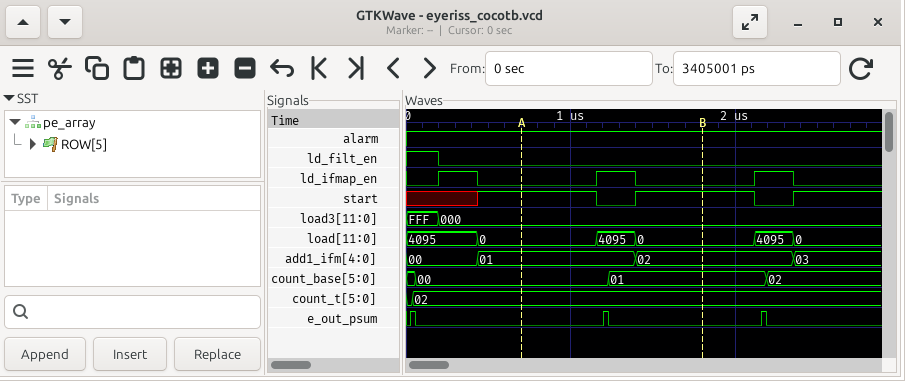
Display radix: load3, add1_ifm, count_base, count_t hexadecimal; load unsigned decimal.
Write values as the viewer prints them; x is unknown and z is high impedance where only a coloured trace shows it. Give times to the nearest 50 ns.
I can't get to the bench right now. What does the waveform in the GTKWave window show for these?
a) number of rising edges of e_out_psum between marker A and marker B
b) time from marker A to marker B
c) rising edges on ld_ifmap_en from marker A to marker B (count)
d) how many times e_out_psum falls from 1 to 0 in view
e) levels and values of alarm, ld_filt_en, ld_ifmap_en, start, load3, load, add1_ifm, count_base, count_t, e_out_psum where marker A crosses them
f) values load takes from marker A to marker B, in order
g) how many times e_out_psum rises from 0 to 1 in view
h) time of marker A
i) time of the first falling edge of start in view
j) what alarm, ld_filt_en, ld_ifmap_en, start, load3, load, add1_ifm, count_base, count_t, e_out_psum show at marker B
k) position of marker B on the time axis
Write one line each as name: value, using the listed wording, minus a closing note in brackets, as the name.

number of rising edges of e_out_psum between marker A and marker B: 1
time from marker A to marker B: 1100 ns
rising edges on ld_ifmap_en from marker A to marker B: 1
how many times e_out_psum falls from 1 to 0 in view: 3
levels and values of alarm, ld_filt_en, ld_ifmap_en, start, load3, load, add1_ifm, count_base, count_t, e_out_psum where marker A crosses them: alarm=1, ld_filt_en=0, ld_ifmap_en=0, start=1, load3=000, load=0, add1_ifm=01, count_base=00, count_t=02, e_out_psum=0
values load takes from marker A to marker B, in order: 0, 4095, 0
how many times e_out_psum rises from 0 to 1 in view: 3
time of marker A: 700 ns
time of the first falling edge of start in view: 1150 ns
what alarm, ld_filt_en, ld_ifmap_en, start, load3, load, add1_ifm, count_base, count_t, e_out_psum show at marker B: alarm=1, ld_filt_en=0, ld_ifmap_en=0, start=1, load3=000, load=0, add1_ifm=02, count_base=01, count_t=02, e_out_psum=0
position of marker B on the time axis: 1800 ns
